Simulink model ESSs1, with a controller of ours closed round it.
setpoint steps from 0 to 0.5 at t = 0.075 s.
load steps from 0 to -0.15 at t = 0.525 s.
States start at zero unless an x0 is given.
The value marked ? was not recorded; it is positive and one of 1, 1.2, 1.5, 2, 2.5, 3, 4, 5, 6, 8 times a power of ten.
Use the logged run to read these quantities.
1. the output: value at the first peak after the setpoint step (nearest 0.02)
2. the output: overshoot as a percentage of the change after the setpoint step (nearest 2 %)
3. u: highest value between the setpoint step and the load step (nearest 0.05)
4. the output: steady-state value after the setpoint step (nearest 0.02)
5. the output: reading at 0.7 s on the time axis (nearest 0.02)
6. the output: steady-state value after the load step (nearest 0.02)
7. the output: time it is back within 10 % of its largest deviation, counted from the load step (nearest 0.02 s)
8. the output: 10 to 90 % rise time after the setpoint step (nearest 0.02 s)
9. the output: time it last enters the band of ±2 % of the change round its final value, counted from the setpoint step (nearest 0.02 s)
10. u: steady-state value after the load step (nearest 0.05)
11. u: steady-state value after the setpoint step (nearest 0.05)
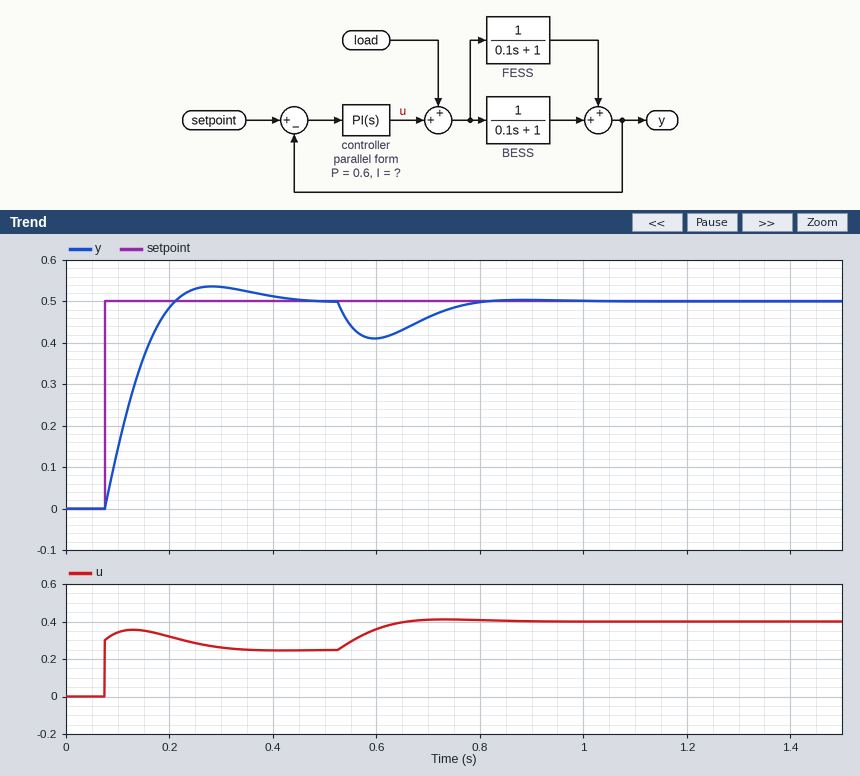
0.54
8 %
0.35
0.50
0.46
0.50
0.24 s
0.10 s
0.34 s
0.40
0.25
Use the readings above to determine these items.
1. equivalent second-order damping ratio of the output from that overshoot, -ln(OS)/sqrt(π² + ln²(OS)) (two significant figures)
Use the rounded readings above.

0.63
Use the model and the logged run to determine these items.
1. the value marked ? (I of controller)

12
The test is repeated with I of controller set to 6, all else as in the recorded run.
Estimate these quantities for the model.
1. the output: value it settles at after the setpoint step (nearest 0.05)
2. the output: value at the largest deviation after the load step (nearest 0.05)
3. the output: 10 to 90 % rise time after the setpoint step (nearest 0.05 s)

0.50
0.40
0.20 s
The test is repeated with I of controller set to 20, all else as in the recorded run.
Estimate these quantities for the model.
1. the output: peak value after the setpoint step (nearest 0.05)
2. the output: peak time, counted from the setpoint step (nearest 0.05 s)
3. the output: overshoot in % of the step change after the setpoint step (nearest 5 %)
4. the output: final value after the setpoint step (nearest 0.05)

0.60
0.15 s
15 %
0.50
